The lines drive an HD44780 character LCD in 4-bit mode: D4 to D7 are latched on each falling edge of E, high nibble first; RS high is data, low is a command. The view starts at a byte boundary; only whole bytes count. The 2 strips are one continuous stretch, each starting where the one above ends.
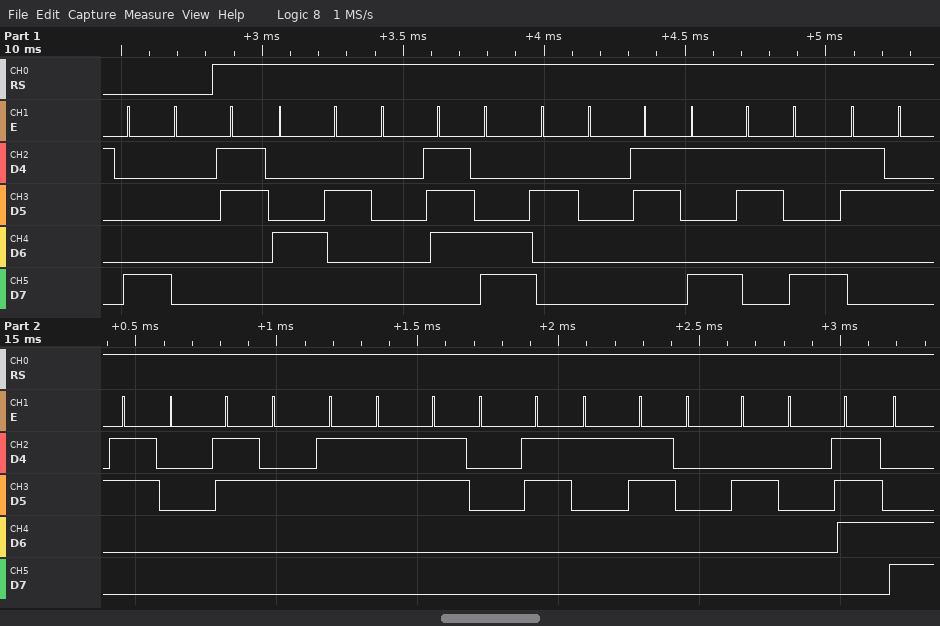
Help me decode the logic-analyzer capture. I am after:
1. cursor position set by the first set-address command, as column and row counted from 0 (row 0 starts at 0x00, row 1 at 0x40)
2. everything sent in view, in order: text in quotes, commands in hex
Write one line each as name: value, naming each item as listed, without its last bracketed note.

cursor position set by the first set-address command, as column and row counted from 0: column 0, row 0
everything sent in view, in order: text in quotes, commands in hex: 0x80 "4 | 992023010 |"
